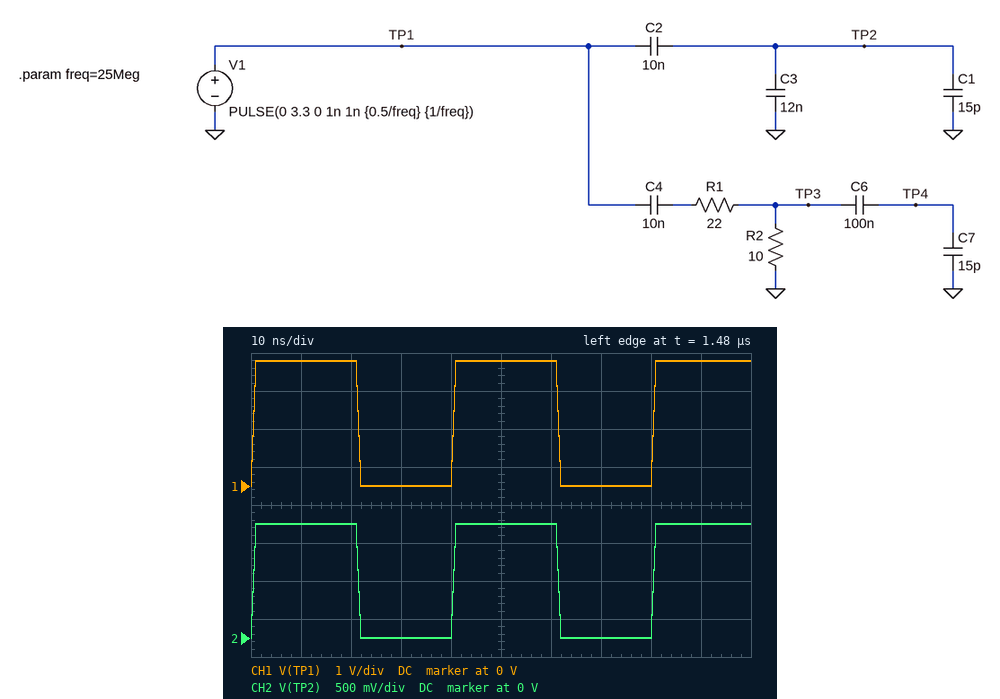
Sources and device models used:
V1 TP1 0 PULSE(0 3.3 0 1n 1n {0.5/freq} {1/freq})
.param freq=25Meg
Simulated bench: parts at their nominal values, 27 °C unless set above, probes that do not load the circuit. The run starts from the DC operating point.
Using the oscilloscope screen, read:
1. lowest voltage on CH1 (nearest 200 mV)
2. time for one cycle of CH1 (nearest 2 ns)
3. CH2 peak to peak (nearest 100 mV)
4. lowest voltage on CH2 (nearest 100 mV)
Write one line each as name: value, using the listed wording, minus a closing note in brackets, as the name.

lowest voltage on CH1: 0 V
time for one cycle of CH1: 40 ns
CH2 peak to peak: 1.5 V
lowest voltage on CH2: 0 V
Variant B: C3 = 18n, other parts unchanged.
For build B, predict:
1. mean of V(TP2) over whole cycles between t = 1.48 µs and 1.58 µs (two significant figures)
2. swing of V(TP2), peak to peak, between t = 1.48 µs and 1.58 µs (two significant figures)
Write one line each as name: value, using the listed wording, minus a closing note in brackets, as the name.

mean of V(TP2) over whole cycles between t = 1.48 µs and 1.58 µs: 620 mV
swing of V(TP2), peak to peak, between t = 1.48 µs and 1.58 µs: 1.2 V
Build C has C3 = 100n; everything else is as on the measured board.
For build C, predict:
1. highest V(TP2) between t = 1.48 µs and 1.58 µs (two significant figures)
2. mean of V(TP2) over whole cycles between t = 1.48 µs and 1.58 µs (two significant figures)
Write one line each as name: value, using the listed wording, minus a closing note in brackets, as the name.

highest V(TP2) between t = 1.48 µs and 1.58 µs: 300 mV
mean of V(TP2) over whole cycles between t = 1.48 µs and 1.58 µs: 160 mV
